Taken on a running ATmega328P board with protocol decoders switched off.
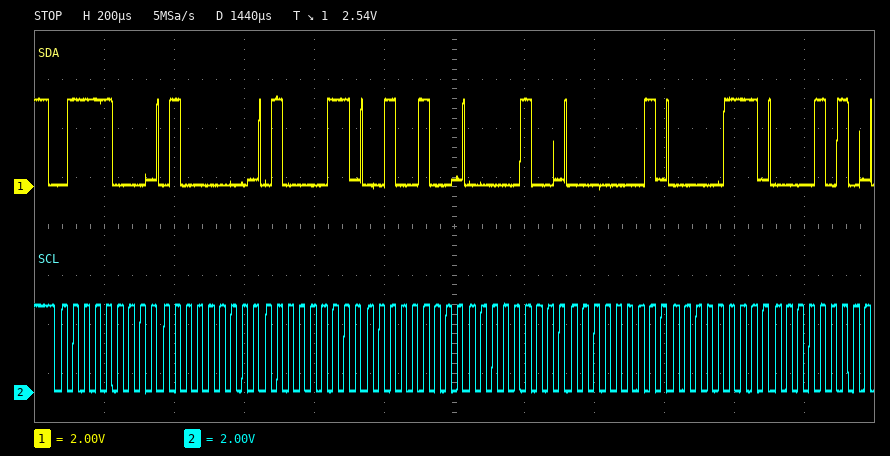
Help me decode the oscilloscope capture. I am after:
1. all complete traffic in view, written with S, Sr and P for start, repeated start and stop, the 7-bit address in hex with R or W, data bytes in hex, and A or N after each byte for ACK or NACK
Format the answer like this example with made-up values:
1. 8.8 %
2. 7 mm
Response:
1. S 3CW A 40 A 43 A 24 A 04 A 01 A 07 A 0A A
